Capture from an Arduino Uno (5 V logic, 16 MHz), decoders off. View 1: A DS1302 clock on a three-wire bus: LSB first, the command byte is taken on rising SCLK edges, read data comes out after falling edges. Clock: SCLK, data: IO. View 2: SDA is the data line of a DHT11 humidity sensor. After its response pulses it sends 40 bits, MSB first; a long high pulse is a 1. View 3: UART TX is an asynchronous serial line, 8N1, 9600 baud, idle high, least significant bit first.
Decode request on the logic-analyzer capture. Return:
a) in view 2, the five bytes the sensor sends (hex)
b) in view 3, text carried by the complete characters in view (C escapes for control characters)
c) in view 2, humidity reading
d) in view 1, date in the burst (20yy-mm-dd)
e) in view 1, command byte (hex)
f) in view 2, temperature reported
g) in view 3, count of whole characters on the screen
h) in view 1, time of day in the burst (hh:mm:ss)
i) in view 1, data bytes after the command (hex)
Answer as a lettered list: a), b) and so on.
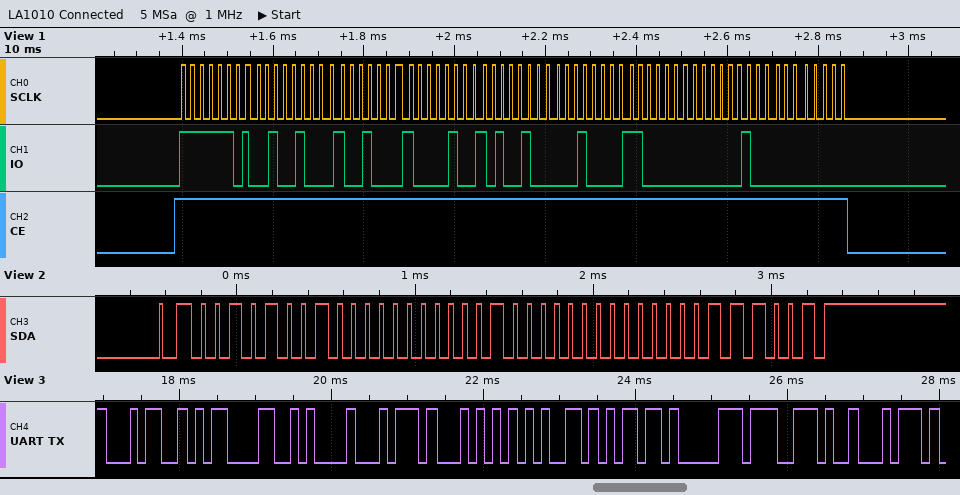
a) 29 00 10 00 39
b) "4\r\ntTemp.t"
c) 41 %
d) 2020-08-25
e) 0xBF
f) 16.0 °C
g) 10
h) 21:12:24
i) 24 12 21 25 08 03 20 00
